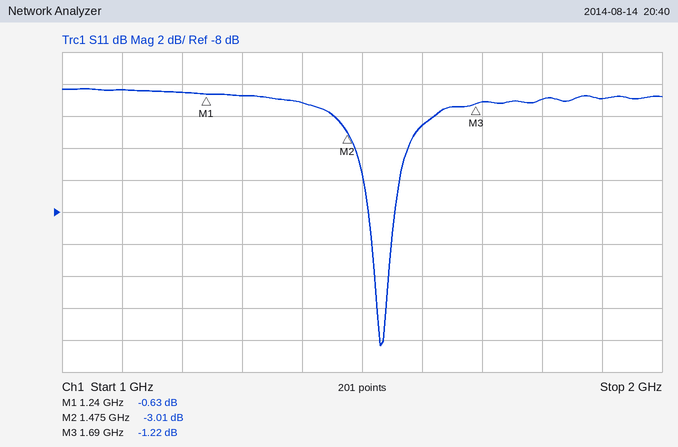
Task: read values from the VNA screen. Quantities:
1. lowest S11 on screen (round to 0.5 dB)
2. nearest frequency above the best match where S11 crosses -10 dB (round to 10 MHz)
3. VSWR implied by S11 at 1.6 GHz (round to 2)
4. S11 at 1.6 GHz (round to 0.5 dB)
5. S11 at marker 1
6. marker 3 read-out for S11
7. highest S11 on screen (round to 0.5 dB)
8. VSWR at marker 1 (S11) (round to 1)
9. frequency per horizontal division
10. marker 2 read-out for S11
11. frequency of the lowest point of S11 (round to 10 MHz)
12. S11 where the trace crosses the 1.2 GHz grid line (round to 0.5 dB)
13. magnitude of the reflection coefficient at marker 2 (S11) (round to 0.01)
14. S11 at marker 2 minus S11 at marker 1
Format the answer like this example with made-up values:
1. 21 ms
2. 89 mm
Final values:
1. -16.5 dB
2. 1.55 GHz
3. 6
4. -2.5 dB
5. -0.63 dB
6. -1.22 dB
7. -0.5 dB
8. 28
9. 100 MHz
10. -3.01 dB
11. 1.53 GHz
12. -0.5 dB
13. 0.71
14. -2.38 dB
